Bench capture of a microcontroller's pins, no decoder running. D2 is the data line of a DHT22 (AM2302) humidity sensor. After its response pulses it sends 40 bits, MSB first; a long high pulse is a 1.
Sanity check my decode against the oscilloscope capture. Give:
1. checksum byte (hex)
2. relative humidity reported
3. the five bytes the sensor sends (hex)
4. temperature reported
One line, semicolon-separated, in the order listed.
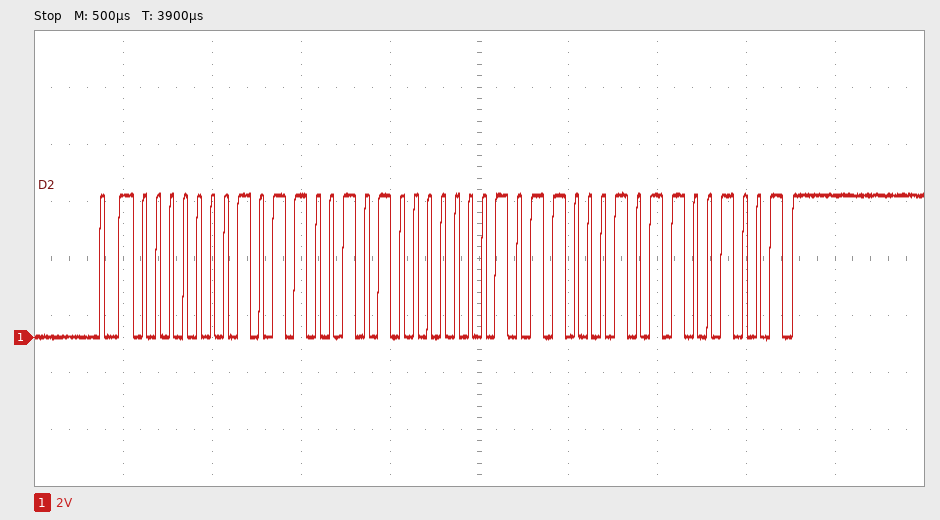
0xC9; 35.7 %; 01 65 01 62 C9; 35.4 °C
